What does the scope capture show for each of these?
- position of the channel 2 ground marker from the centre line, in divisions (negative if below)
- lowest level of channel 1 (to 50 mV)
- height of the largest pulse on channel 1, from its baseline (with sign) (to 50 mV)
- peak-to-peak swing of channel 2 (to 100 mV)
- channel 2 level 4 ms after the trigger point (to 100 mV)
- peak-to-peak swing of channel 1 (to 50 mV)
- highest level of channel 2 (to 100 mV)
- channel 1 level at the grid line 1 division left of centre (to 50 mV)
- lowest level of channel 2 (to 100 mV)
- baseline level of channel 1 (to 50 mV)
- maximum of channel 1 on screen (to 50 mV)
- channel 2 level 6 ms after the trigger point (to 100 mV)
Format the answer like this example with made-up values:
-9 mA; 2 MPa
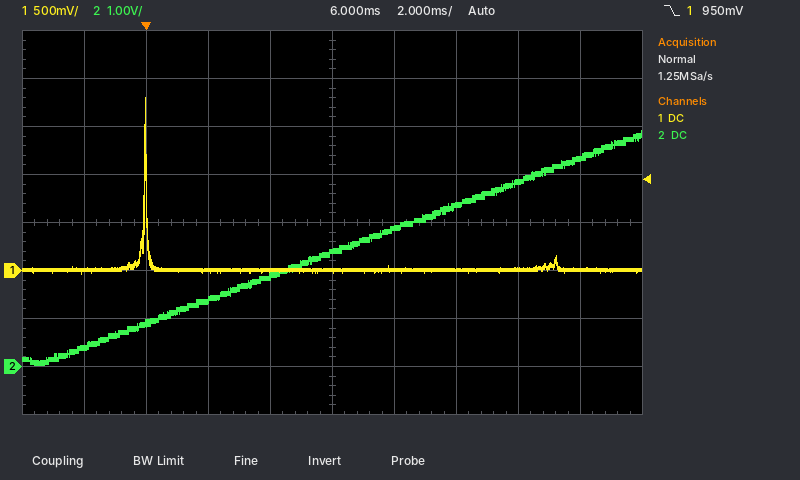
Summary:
-3.0 div; -50 mV; +1.80 V; 4.9 V; 1.9 V; 1.85 V; 4.9 V; 0 mV; 0.0 V; 0 mV; 1.80 V; 2.4 V
